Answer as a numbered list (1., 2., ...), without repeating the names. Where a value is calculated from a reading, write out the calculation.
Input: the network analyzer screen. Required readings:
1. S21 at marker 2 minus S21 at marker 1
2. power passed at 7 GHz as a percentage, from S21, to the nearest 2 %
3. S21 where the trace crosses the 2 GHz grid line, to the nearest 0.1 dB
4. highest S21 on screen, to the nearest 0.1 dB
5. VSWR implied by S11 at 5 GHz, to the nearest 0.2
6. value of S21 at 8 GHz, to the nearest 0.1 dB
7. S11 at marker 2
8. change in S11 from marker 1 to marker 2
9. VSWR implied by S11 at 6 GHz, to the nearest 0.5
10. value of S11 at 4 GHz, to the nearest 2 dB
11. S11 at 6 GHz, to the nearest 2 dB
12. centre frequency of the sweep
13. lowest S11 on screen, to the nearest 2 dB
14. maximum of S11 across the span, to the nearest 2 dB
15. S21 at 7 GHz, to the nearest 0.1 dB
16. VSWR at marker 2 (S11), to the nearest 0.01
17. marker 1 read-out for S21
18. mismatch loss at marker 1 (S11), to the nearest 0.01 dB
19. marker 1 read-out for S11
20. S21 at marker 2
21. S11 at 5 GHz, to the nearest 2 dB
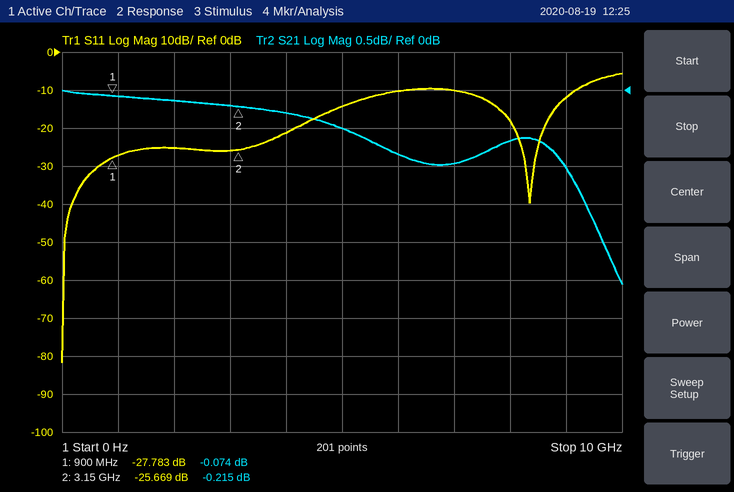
1. -0.215 − (-0.074) = -0.141 dB
2. 10^(-1/10) ≈ 79.4 %, so 80 % to the nearest 2 %
3. -0.1 dB
4. 0.0 dB
5. |Γ| = 10^(-14/20) = 0.1995; VSWR = (1 + 0.1995)/(1 − 0.1995) ≈ 1.50, so 1.4 to the nearest 0.2
6. -0.7 dB
7. -25.669 dB
8. -25.669 − (-27.783) = 2.114 dB
9. |Γ| = 10^(-10/20) = 0.3162; VSWR = (1 + 0.3162)/(1 − 0.3162) ≈ 1.92, so 2.0 to the nearest 0.5
10. -22 dB
11. -10 dB
12. 5 GHz
13. -82 dB
14. -6 dB
15. -1.0 dB
16. (1 + 0.0521)/(1 − 0.0521) ≈ 1.11
17. -0.074 dB
18. −10 log10(1 − 10^(-27.783/10)) ≈ 0.01 dB
19. -27.783 dB
20. -0.215 dB
21. -14 dB
